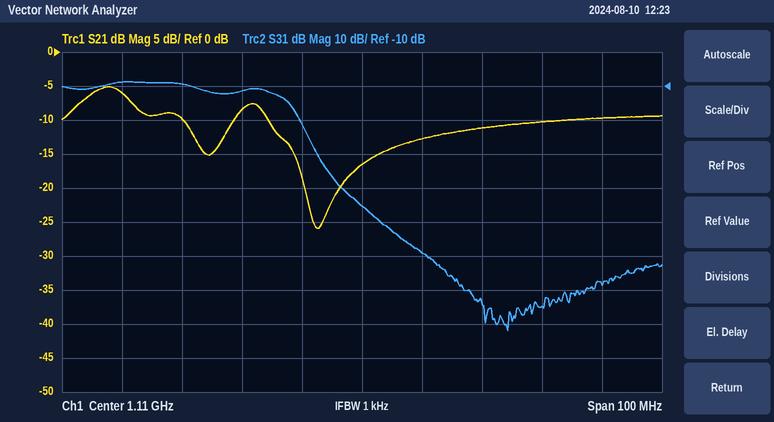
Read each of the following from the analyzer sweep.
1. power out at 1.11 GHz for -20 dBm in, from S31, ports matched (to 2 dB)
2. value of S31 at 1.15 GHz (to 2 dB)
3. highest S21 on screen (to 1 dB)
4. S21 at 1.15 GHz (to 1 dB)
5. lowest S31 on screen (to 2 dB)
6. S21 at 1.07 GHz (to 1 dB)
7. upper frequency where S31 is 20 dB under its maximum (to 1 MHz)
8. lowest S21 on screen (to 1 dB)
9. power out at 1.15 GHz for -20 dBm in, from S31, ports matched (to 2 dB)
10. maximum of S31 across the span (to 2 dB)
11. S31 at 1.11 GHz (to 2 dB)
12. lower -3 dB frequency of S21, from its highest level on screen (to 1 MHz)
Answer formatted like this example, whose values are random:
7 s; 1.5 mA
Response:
-66 dBm; -68 dB; -5 dB; -10 dB; -82 dB; -6 dB; 1.102 GHz; -26 dB; -88 dBm; -8 dB; -46 dB; 1.062 GHz
